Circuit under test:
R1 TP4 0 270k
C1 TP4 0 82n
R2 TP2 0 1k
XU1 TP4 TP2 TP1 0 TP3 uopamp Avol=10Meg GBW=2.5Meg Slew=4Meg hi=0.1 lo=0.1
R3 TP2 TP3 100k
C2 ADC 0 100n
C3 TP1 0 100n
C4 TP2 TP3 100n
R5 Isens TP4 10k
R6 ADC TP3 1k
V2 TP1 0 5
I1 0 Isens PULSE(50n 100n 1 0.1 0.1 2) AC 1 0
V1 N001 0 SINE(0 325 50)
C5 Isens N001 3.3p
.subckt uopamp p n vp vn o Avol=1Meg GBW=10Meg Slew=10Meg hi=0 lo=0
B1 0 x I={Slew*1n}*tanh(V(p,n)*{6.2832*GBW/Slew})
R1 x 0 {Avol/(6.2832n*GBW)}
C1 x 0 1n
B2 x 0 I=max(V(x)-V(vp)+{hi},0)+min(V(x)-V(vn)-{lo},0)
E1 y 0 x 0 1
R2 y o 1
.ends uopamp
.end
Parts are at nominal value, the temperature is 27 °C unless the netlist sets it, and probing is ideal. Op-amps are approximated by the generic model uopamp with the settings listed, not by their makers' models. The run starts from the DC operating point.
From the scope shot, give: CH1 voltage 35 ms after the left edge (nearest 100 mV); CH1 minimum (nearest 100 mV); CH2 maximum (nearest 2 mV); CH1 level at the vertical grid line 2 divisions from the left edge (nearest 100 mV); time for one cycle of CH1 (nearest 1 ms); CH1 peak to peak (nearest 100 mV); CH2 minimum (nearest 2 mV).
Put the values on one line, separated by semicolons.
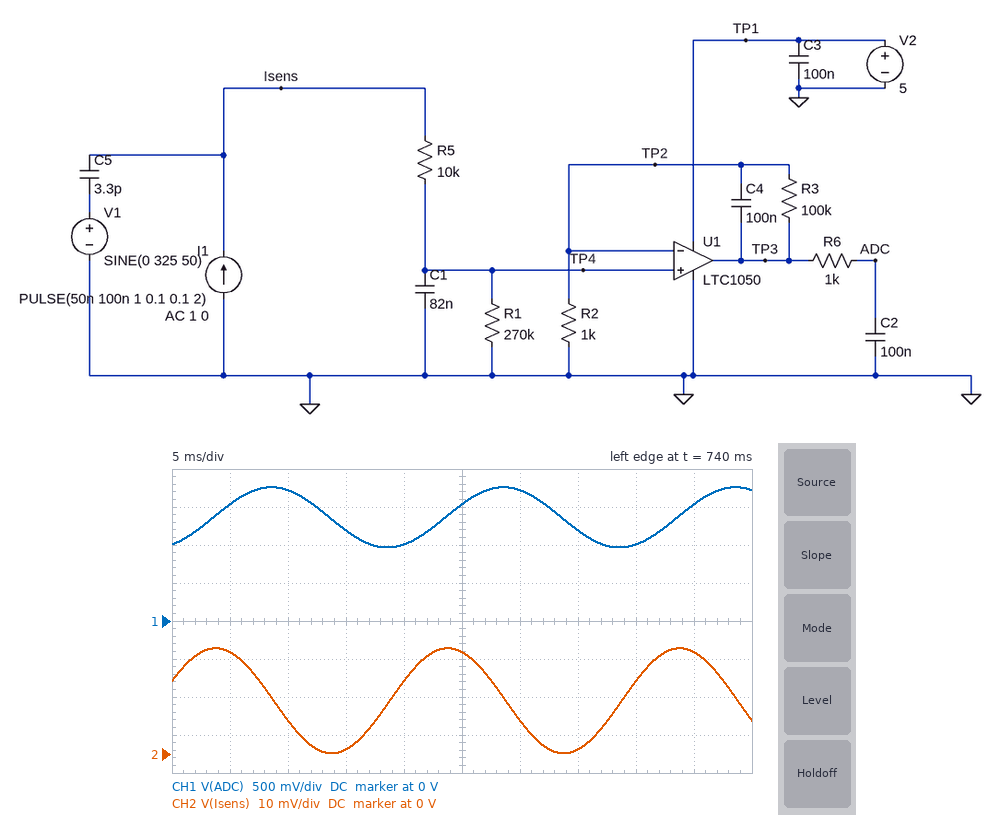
1.2 V; 1.0 V; 28 mV; 1.7 V; 20 ms; 800 mV; 0 V
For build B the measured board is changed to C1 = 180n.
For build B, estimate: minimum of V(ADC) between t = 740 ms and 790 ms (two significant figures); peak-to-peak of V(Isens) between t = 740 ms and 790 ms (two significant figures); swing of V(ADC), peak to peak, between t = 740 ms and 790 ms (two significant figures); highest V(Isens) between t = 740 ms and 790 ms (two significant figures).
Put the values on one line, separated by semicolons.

1.2 V; 14 mV; 360 mV; 21 mV
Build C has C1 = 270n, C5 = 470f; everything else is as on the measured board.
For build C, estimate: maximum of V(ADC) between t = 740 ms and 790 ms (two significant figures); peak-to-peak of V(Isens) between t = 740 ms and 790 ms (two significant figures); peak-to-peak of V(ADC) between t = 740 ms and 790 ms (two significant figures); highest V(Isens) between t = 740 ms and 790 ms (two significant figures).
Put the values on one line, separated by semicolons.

1.4 V; 1.5 mV; 35 mV; 15 mV
